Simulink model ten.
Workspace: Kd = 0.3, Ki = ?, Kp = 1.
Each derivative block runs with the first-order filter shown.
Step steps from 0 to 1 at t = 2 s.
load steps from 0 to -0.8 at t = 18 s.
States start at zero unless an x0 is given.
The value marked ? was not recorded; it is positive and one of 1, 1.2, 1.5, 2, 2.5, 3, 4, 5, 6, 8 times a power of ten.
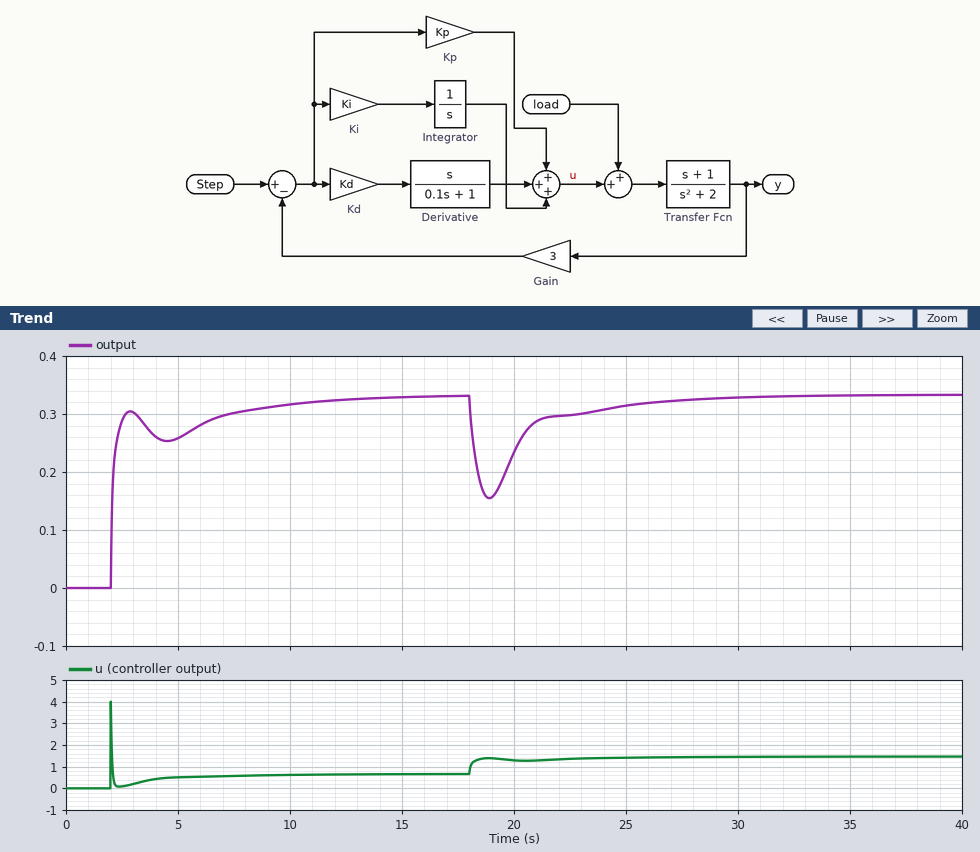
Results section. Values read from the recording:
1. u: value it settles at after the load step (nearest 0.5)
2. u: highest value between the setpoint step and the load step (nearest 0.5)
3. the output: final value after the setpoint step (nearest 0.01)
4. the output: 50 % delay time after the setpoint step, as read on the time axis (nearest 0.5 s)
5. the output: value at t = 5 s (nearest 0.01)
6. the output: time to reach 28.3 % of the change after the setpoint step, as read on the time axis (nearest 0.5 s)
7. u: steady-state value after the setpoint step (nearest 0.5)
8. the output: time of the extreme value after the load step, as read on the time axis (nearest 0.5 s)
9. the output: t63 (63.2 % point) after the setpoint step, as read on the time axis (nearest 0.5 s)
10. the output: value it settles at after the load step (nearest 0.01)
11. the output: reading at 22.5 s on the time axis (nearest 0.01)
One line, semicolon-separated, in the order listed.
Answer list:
1.5; 4.0; 0.33; 2.0 s; 0.26; 2.0 s; 0.5; 19.0 s; 2.0 s; 0.33; 0.30
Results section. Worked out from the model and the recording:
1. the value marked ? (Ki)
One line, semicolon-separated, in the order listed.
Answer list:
0.5
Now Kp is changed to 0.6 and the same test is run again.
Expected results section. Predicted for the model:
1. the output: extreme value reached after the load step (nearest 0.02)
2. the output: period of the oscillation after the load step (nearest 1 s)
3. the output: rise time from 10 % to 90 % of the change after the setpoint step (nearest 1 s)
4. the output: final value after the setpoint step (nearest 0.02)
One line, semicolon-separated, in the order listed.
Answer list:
0.10; 4 s; 5 s; 0.34
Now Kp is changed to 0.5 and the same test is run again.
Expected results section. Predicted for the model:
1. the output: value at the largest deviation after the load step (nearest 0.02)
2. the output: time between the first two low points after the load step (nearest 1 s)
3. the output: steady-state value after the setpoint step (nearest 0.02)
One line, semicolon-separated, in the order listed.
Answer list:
0.08; 4 s; 0.34
